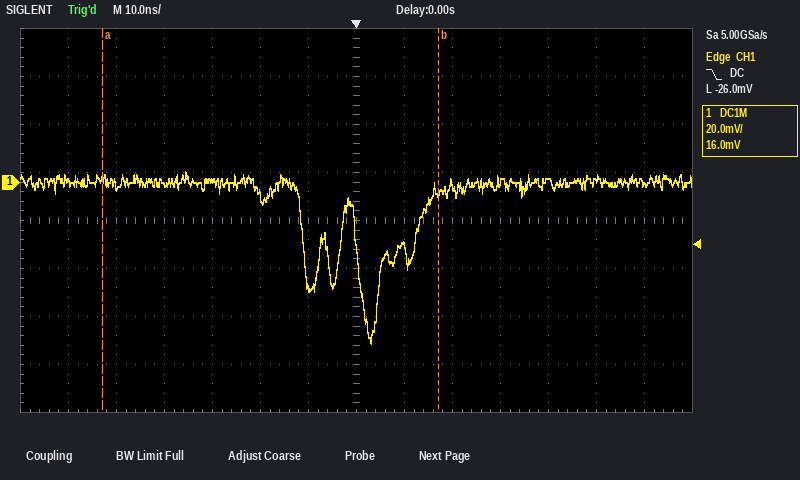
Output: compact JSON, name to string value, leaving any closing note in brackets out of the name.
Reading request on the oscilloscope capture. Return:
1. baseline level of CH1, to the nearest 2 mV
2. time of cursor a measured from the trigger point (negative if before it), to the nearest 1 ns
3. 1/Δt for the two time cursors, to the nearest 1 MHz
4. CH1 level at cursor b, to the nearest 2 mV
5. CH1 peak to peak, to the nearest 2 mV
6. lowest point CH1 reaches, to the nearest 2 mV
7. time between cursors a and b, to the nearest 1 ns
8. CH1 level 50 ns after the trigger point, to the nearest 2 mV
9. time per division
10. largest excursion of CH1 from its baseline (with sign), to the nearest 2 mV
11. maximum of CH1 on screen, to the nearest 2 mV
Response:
{"baseline level of CH1, to the nearest 2 mV": "0 mV", "time of cursor a measured from the trigger point (negative if before it), to the nearest 1 ns": "-53 ns", "1/Δt for the two time cursors, to the nearest 1 MHz": "14 MHz", "CH1 level at cursor b, to the nearest 2 mV": "-4 mV", "CH1 peak to peak, to the nearest 2 mV": "72 mV", "lowest point CH1 reaches, to the nearest 2 mV": "-68 mV", "time between cursors a and b, to the nearest 1 ns": "70 ns", "CH1 level 50 ns after the trigger point, to the nearest 2 mV": "2 mV", "time per division": "10 ns", "largest excursion of CH1 from its baseline (with sign), to the nearest 2 mV": "-68 mV", "maximum of CH1 on screen, to the nearest 2 mV": "4 mV"}
